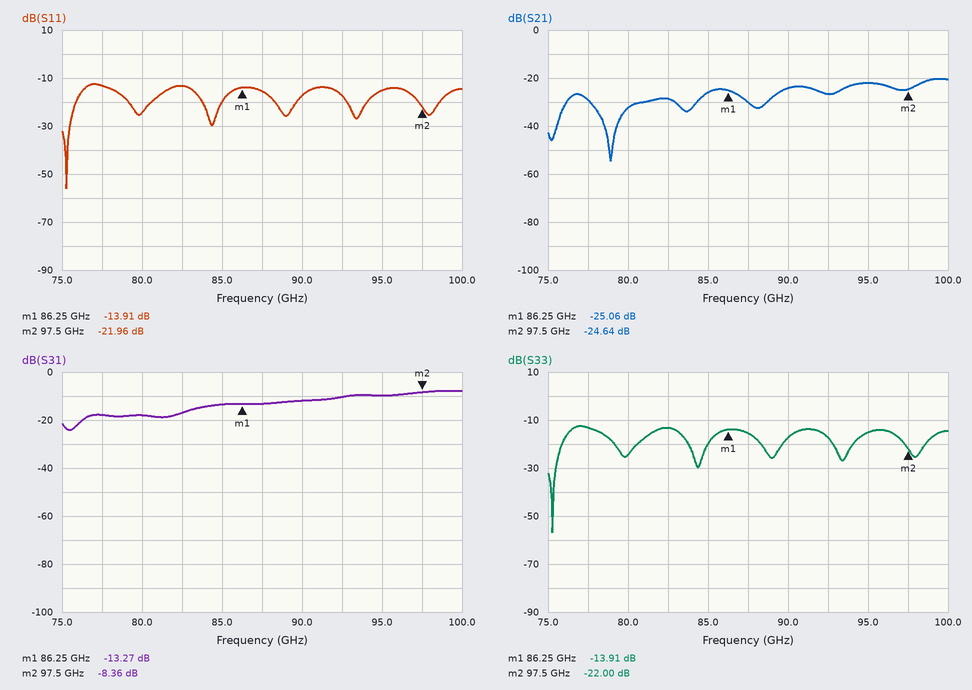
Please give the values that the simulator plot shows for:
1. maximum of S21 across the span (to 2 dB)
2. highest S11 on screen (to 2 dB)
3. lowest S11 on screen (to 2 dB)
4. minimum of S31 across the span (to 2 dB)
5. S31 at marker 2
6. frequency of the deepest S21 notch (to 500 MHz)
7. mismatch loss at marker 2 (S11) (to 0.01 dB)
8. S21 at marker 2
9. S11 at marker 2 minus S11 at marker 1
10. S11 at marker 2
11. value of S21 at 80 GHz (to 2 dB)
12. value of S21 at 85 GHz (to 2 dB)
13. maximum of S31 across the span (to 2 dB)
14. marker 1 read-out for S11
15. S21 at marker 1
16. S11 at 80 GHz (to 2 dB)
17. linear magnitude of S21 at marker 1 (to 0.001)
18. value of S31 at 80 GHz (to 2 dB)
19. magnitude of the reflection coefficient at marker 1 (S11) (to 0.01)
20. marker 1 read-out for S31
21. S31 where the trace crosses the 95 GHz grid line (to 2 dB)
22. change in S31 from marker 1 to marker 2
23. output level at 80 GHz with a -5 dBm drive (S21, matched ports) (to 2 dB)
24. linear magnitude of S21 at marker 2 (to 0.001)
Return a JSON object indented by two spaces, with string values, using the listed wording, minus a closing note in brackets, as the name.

{
  "maximum of S21 across the span": "-20 dB",
  "highest S11 on screen": "-12 dB",
  "lowest S11 on screen": "-56 dB",
  "minimum of S31 across the span": "-24 dB",
  "S31 at marker 2": "-8.36 dB",
  "frequency of the deepest S21 notch": "79.0 GHz",
  "mismatch loss at marker 2 (S11)": "0.03 dB",
  "S21 at marker 2": "-24.64 dB",
  "S11 at marker 2 minus S11 at marker 1": "-8.05 dB",
  "S11 at marker 2": "-21.96 dB",
  "value of S21 at 80 GHz": "-32 dB",
  "value of S21 at 85 GHz": "-26 dB",
  "maximum of S31 across the span": "-8 dB",
  "marker 1 read-out for S11": "-13.91 dB",
  "S21 at marker 1": "-25.06 dB",
  "S11 at 80 GHz": "-24 dB",
  "linear magnitude of S21 at marker 1": "0.056",
  "value of S31 at 80 GHz": "-18 dB",
  "magnitude of the reflection coefficient at marker 1 (S11)": "0.20",
  "marker 1 read-out for S31": "-13.27 dB",
  "S31 where the trace crosses the 95 GHz grid line": "-10 dB",
  "change in S31 from marker 1 to marker 2": "4.91 dB",
  "output level at 80 GHz with a -5 dBm drive (S21, matched ports)": "-38 dBm",
  "linear magnitude of S21 at marker 2": "0.059"
}
